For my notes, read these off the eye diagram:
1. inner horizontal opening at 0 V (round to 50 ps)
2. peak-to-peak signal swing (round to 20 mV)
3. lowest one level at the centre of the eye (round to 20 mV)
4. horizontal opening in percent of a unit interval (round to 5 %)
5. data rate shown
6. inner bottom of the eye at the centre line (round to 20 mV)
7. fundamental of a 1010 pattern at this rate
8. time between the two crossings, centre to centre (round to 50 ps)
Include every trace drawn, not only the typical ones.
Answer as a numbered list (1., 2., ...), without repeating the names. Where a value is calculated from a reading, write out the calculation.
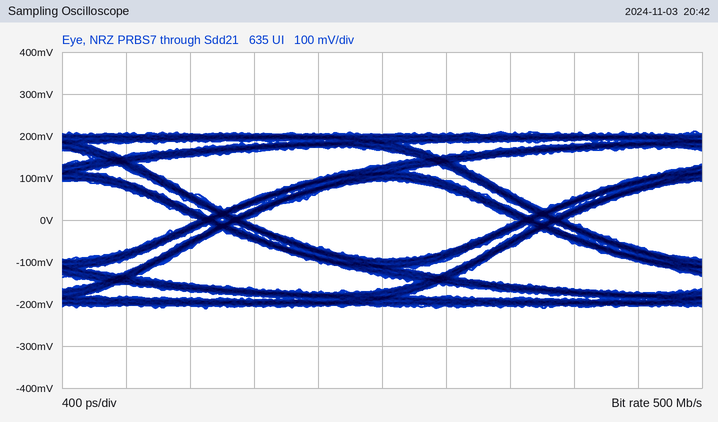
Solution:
1. 1.70 ns
2. 420 mV
3. 100 mV
4. 1.70 ns / 2.00 ns ≈ 85 %
5. 500 Mb/s
6. -100 mV
7. 250 MHz
8. 2.00 ns
